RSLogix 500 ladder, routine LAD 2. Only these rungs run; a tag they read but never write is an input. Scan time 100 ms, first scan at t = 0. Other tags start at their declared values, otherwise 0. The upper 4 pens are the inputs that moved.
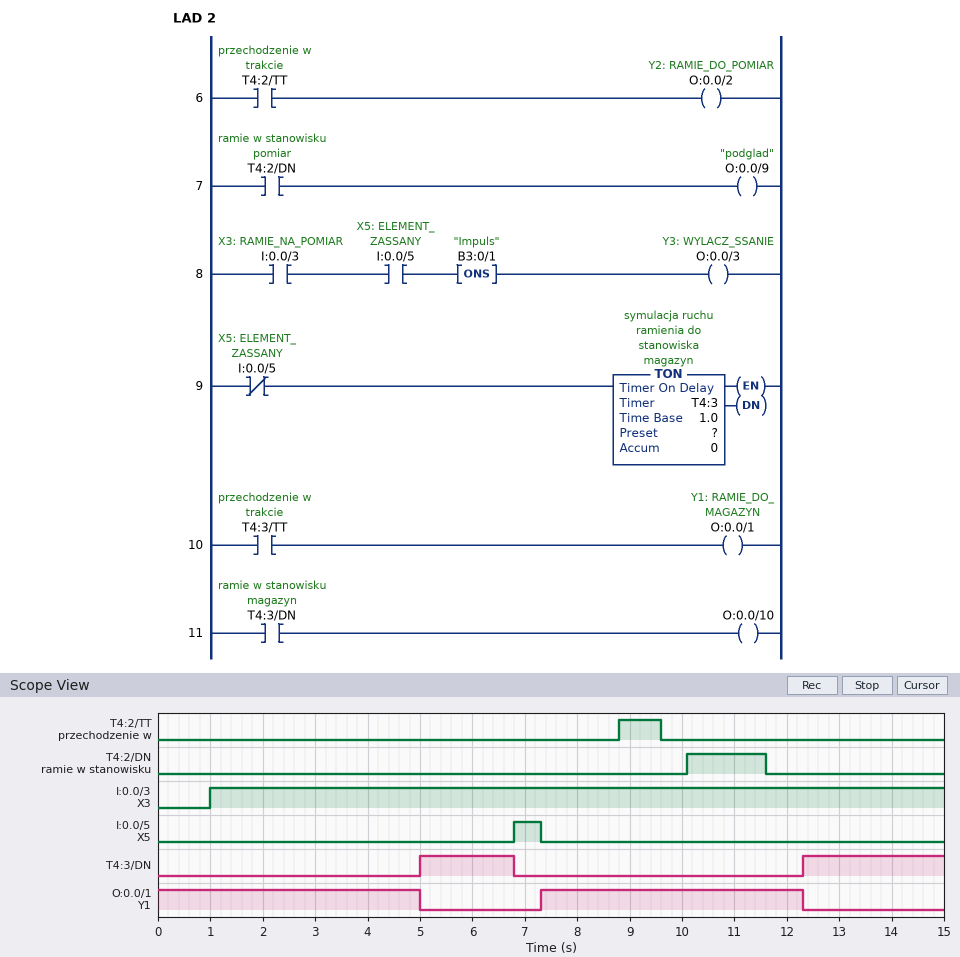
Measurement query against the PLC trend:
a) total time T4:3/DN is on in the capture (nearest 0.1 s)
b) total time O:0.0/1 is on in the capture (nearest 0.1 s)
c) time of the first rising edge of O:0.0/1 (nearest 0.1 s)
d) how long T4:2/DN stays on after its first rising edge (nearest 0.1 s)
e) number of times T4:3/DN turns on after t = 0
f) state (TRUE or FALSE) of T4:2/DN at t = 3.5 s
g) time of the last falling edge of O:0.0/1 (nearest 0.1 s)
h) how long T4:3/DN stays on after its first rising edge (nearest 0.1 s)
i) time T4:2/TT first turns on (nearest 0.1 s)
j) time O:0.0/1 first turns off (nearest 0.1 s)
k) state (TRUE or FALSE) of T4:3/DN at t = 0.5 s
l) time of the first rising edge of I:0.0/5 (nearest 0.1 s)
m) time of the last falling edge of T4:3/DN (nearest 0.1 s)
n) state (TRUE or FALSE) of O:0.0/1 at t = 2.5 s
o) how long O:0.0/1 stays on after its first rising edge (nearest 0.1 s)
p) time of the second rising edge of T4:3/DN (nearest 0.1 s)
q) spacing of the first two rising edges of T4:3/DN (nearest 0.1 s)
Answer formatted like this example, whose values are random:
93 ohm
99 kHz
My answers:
4.5 s
10.0 s
7.3 s
1.5 s
2
FALSE
12.3 s
1.8 s
8.8 s
5.0 s
FALSE
6.8 s
6.8 s
TRUE
5.0 s
12.3 s
7.3 s
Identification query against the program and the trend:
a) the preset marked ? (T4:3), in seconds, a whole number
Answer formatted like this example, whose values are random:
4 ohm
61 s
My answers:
5 s
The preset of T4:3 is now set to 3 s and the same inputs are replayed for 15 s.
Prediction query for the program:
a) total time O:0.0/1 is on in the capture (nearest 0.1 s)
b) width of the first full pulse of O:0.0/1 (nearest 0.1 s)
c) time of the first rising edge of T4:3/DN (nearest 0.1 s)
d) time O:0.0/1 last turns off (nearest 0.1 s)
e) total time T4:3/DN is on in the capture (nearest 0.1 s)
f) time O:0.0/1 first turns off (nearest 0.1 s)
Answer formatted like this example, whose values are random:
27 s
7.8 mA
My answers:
6.0 s
3.0 s
3.0 s
10.3 s
8.5 s
3.0 s
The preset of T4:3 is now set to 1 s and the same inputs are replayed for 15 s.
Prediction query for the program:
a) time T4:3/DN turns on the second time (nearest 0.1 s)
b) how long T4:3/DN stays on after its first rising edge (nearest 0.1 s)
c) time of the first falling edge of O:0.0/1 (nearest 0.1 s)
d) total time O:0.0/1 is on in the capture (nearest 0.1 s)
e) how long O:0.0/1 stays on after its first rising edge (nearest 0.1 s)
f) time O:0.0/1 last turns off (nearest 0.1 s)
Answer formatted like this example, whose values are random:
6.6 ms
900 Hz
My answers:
8.3 s
5.8 s
1.0 s
2.0 s
1.0 s
8.3 s
